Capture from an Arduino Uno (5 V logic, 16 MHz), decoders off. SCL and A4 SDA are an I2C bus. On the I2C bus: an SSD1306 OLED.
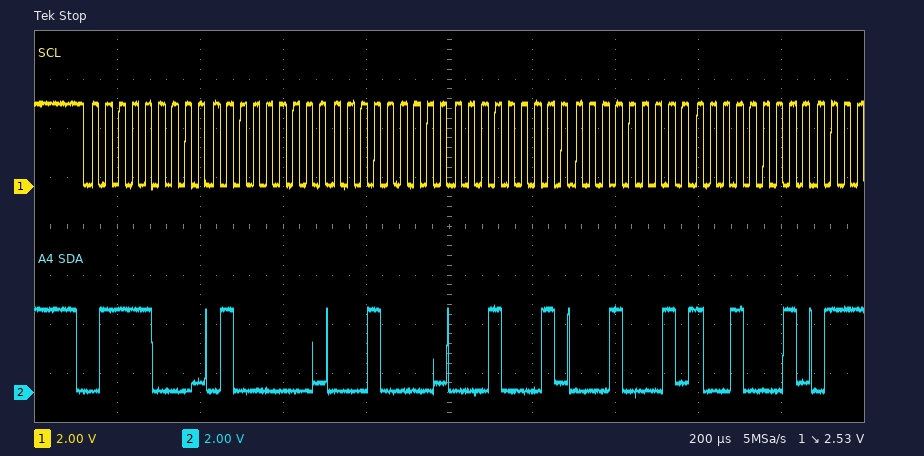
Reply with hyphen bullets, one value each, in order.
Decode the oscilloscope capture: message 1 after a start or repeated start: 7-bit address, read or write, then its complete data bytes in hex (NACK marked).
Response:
- 0x3C write: 40 10 11 11 91
